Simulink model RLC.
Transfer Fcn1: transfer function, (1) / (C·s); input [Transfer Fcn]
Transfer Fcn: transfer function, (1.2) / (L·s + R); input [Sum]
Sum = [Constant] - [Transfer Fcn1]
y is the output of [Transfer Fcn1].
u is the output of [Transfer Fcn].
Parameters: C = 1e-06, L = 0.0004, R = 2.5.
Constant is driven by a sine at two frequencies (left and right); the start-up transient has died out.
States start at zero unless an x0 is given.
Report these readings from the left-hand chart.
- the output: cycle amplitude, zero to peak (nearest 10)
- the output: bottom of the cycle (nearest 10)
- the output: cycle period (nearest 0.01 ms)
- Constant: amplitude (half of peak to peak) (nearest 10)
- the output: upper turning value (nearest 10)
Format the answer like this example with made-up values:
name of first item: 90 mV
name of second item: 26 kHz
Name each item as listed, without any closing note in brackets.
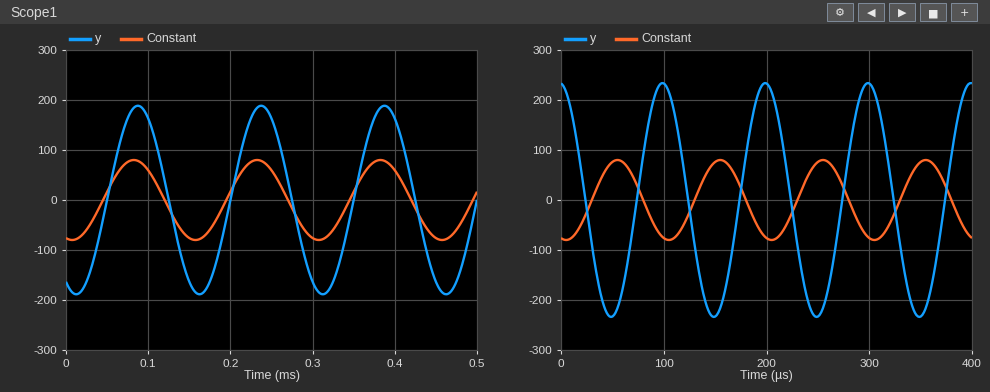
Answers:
the output: cycle amplitude, zero to peak: 190
the output: bottom of the cycle: -190
the output: cycle period: 0.15 ms
Constant: amplitude (half of peak to peak): 80
the output: upper turning value: 190
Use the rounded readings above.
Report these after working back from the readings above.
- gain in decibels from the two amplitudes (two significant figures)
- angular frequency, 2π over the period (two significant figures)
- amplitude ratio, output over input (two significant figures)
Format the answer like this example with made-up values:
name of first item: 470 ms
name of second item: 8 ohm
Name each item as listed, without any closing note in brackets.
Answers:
gain in decibels from the two amplitudes: 7.5 dB
angular frequency, 2π over the period: 42 rad/ms
amplitude ratio, output over input: 2.4
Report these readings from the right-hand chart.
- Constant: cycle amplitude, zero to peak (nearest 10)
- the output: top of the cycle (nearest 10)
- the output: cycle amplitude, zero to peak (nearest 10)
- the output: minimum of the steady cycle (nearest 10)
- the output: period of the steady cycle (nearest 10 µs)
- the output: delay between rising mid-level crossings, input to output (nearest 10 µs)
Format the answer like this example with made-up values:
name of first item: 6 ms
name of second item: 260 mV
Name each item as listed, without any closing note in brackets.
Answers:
Constant: cycle amplitude, zero to peak: 80
the output: top of the cycle: 230
the output: cycle amplitude, zero to peak: 230
the output: minimum of the steady cycle: -230
the output: period of the steady cycle: 100 µs
the output: delay between rising mid-level crossings, input to output: 40 µs
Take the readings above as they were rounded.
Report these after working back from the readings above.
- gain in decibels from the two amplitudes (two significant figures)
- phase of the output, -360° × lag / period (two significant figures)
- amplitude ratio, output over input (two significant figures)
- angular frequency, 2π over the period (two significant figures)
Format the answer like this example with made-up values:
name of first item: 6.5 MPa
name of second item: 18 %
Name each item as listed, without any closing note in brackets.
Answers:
gain in decibels from the two amplitudes: 9.2 dB
phase of the output, -360° × lag / period: -140°
amplitude ratio, output over input: 2.9
angular frequency, 2π over the period: 0.063 rad/µs
